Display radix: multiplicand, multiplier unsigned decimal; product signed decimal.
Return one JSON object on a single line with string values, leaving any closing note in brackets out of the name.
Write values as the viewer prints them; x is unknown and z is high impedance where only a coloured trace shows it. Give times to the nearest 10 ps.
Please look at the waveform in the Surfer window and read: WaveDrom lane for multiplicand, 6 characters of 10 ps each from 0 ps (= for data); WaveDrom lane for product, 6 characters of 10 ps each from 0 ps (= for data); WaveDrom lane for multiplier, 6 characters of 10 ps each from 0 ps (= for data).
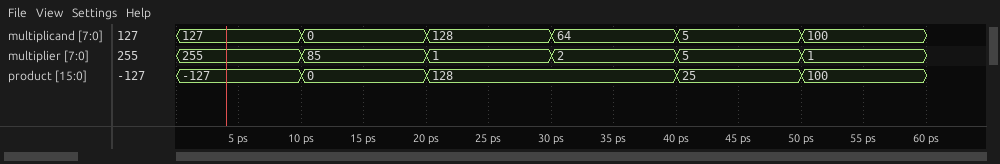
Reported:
{"WaveDrom lane for multiplicand, 6 characters of 10 ps each from 0 ps": "{name: 'multiplicand', wave: '======', data: '127 0 128 64 5 100'}", "WaveDrom lane for product, 6 characters of 10 ps each from 0 ps": "{name: 'product', wave: '===.==', data: '-127 0 128 25 100'}", "WaveDrom lane for multiplier, 6 characters of 10 ps each from 0 ps": "{name: 'multiplier', wave: '======', data: '255 85 1 2 5 1'}"}
